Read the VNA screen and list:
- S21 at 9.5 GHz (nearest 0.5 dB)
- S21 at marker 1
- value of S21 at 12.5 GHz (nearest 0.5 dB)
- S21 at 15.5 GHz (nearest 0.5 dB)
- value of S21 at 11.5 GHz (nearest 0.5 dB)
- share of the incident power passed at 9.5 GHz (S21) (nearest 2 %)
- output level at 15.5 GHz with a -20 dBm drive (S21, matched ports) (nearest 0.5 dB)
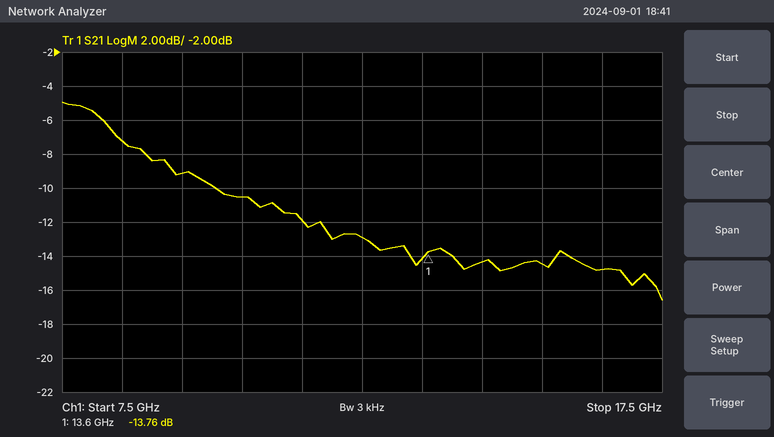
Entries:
-9.0 dB
-13.76 dB
-13.0 dB
-14.5 dB
-12.0 dB
12 %
-34.5 dBm
